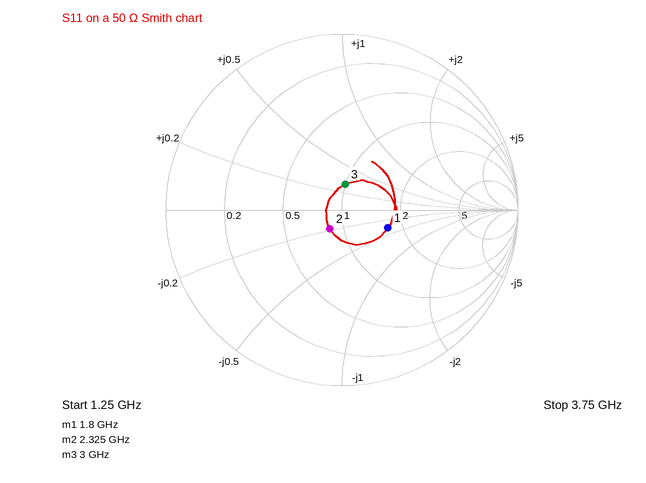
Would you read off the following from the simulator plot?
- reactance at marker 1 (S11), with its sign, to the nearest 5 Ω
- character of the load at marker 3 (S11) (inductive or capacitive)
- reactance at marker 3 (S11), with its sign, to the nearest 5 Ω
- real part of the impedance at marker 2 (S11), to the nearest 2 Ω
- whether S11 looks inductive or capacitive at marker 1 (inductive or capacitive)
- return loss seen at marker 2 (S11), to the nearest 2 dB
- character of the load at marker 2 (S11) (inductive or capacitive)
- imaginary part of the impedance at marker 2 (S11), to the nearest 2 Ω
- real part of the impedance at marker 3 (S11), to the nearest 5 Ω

-20 Ω
inductive
+15 Ω
42 Ω
capacitive
18 dB
capacitive
-10 Ω
50 Ω
